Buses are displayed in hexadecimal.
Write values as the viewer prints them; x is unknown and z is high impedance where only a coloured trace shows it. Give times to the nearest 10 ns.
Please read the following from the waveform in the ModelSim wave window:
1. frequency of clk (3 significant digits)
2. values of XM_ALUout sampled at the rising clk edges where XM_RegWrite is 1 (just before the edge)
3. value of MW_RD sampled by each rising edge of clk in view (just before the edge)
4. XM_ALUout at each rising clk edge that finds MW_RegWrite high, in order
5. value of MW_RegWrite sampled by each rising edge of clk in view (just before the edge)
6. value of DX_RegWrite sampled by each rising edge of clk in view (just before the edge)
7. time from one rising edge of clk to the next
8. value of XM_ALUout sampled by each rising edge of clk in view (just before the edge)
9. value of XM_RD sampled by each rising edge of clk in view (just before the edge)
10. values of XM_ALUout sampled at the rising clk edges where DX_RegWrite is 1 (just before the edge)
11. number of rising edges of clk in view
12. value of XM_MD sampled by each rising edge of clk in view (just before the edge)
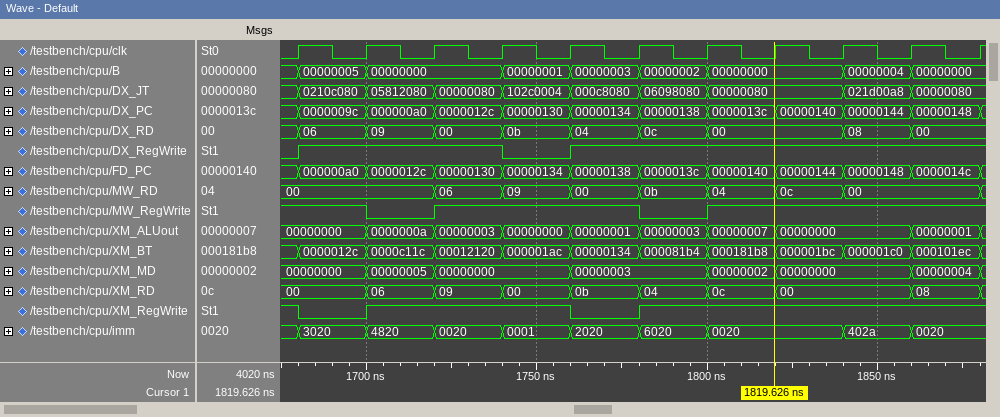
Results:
50.0 MHz
00000000, 0000000a, 00000003, 00000000, 00000003, 00000007, 00000000, 00000000, 00000001
00, 00, 00, 06, 09, 00, 0b, 04, 0c, 00, 00
00000000, 00000000, 00000003, 00000000, 00000001, 00000007, 00000000, 00000000, 00000001
1 1 0 1 1 1 0 1 1 1 1
0 1 1 1 0 1 1 1 1 1 1
20 ns
00000000, 00000000, 0000000a, 00000003, 00000000, 00000001, 00000003, 00000007, 00000000, 00000000, 00000001
00, 00, 06, 09, 00, 0b, 04, 0c, 00, 00, 08
00000000, 0000000a, 00000003, 00000001, 00000003, 00000007, 00000000, 00000000, 00000001
11
00000000, 00000000, 00000005, 00000000, 00000000, 00000003, 00000003, 00000002, 00000000, 00000000, 00000004
